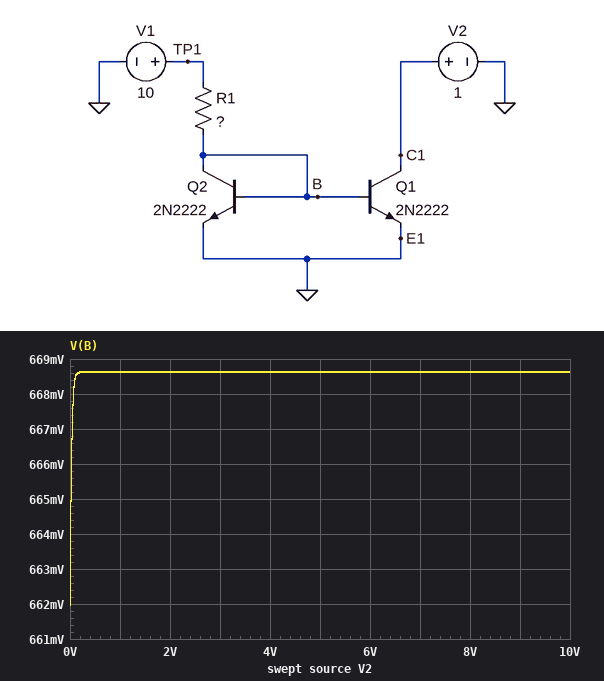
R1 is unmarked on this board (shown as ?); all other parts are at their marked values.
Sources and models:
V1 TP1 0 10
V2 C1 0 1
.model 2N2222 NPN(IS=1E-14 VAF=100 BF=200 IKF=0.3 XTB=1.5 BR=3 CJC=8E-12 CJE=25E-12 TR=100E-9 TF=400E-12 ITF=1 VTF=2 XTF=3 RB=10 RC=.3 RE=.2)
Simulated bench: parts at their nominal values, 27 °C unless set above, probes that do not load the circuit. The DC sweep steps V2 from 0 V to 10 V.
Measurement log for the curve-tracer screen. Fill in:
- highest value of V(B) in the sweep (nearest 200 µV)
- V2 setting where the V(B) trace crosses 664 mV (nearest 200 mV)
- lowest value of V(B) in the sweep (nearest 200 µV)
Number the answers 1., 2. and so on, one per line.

1. 668.6 mV
2. 0 V
3. 662.0 mV
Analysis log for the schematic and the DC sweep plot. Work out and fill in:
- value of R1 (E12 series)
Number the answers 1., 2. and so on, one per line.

1. 5.6 kΩ
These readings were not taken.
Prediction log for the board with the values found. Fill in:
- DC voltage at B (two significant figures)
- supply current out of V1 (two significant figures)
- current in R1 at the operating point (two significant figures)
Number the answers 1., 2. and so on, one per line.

1. 670 mV
2. 1.7 mA
3. 1.7 mA
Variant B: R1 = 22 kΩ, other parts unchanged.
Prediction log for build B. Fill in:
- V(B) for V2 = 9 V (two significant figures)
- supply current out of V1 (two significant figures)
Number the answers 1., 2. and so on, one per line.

1. 630 mV
2. 430 µA
